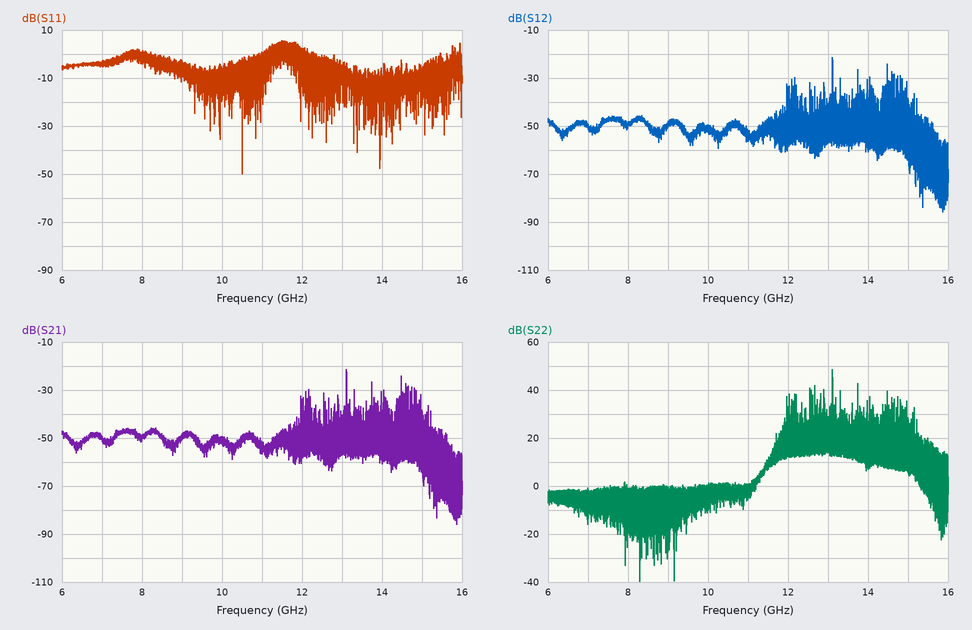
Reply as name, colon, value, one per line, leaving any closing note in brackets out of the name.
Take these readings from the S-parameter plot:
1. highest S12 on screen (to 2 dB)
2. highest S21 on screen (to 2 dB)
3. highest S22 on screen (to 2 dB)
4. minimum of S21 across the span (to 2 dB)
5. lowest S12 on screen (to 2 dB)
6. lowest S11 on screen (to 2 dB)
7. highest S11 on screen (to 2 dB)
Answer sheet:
highest S12 on screen: -22 dB
highest S21 on screen: -22 dB
highest S22 on screen: 48 dB
minimum of S21 across the span: -86 dB
lowest S12 on screen: -86 dB
lowest S11 on screen: -50 dB
highest S11 on screen: 6 dB
